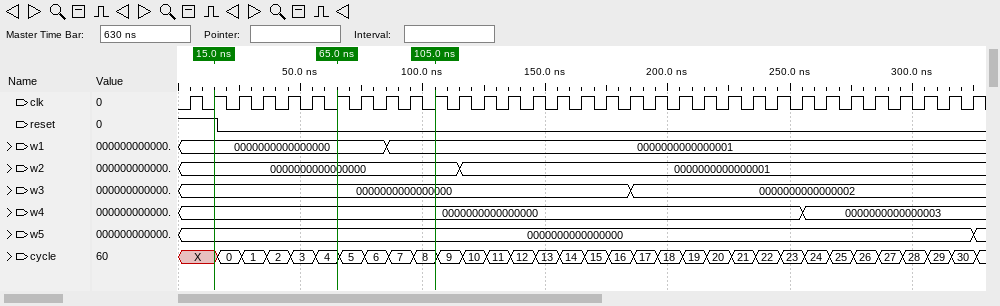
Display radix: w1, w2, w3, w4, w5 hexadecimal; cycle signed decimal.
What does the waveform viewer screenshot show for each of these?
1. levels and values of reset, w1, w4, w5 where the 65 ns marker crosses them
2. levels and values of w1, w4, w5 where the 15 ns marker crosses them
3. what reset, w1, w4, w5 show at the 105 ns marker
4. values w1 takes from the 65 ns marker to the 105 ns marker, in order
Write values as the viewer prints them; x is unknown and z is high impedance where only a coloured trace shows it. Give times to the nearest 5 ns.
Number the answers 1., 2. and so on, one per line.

1. reset=0, w1=0000000000000000, w4=0000000000000000, w5=0000000000000000
2. w1=0000000000000000, w4=0000000000000000, w5=0000000000000000
3. reset=0, w1=0000000000000001, w4=0000000000000000, w5=0000000000000000
4. 0000000000000000, 0000000000000001
